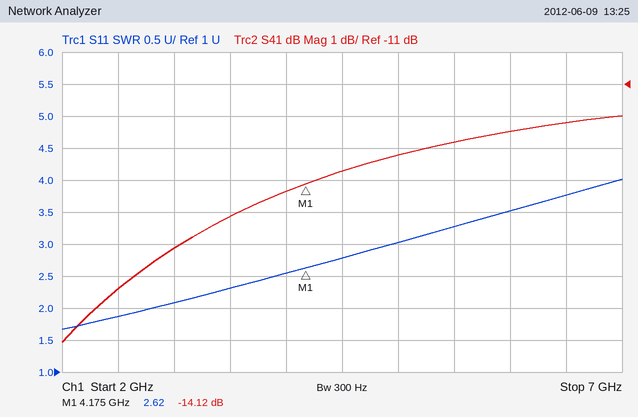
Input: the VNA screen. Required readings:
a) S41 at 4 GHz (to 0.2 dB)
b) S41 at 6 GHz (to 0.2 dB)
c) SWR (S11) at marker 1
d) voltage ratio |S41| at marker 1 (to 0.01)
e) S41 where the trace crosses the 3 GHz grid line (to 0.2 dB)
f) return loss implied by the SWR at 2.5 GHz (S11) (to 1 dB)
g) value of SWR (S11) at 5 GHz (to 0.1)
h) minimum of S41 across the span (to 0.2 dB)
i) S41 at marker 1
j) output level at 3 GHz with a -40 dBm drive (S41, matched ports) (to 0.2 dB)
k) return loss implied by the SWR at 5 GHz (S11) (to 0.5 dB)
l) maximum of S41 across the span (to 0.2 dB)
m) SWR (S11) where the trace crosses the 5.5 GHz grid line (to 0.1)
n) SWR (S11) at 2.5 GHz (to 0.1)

-14.4 dB
-12.4 dB
2.62
0.20
-16.2 dB
10 dB
3.0
-19.0 dB
-14.12 dB
-56.2 dBm
6.0 dB
-12.0 dB
3.3
1.9
